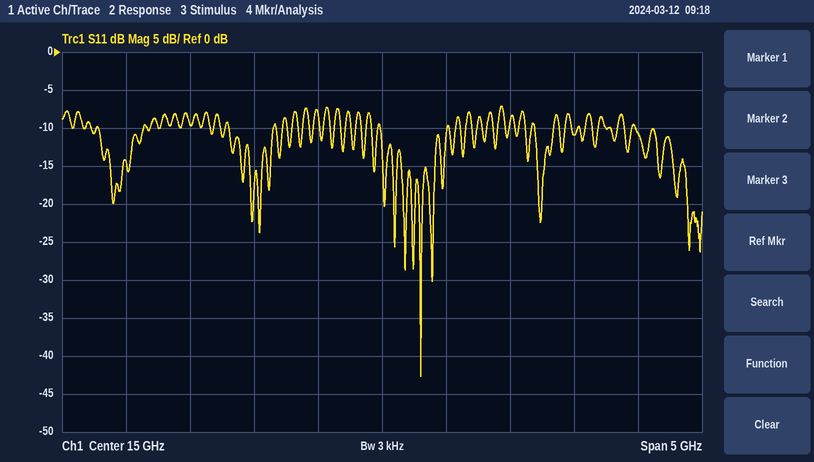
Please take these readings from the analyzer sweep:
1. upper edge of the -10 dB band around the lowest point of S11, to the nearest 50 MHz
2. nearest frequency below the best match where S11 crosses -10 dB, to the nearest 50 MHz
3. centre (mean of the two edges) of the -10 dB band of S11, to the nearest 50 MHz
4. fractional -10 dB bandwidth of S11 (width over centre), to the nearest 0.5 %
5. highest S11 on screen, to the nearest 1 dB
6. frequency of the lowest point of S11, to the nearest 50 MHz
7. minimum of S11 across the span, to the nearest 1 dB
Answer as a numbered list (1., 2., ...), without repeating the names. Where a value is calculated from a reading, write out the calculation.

1. 15.50 GHz
2. 15.00 GHz
3. 15.25 GHz
4. 500 MHz / 15.25 GHz ≈ 3.28 %, so 3.5 % to the nearest 0.5 %
5. -7 dB
6. 15.30 GHz
7. -43 dB
